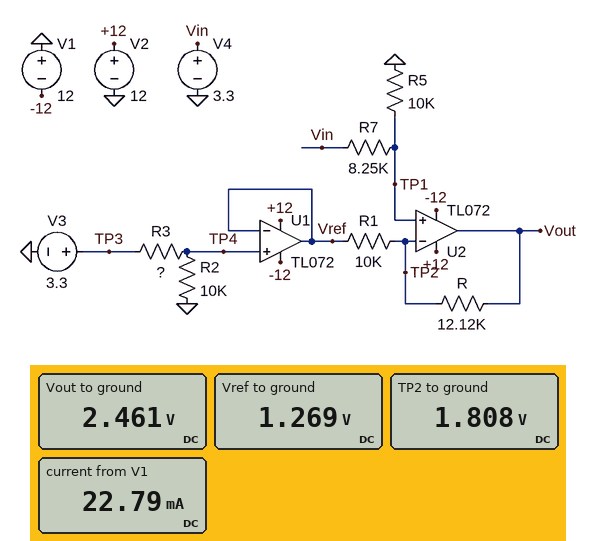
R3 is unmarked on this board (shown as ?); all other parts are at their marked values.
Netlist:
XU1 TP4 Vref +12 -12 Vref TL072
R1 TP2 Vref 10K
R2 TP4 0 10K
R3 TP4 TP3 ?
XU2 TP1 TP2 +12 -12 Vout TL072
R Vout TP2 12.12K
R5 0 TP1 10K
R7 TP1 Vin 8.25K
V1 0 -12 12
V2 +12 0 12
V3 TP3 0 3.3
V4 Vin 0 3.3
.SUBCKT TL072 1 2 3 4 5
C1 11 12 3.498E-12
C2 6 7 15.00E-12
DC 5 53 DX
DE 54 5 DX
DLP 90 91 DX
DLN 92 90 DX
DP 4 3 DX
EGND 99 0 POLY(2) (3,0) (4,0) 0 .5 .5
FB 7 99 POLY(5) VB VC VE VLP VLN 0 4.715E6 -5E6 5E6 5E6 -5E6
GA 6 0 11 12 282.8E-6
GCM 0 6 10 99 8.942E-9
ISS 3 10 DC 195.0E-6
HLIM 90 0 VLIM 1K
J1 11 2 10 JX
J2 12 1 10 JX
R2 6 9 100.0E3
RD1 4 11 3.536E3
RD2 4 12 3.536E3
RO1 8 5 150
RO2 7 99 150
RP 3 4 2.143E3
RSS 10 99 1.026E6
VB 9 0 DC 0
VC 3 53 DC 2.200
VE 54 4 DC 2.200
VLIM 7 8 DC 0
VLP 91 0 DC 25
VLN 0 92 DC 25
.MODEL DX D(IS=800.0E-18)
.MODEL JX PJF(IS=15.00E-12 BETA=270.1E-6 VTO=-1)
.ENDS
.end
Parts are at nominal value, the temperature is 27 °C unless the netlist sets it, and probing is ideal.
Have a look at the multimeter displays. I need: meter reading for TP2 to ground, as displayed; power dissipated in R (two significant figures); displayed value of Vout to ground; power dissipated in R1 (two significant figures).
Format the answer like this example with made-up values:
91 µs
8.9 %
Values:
1.808 V
35 µW
2.461 V
29 µW
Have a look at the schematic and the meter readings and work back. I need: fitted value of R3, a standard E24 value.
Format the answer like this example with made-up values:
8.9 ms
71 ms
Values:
16 kΩ
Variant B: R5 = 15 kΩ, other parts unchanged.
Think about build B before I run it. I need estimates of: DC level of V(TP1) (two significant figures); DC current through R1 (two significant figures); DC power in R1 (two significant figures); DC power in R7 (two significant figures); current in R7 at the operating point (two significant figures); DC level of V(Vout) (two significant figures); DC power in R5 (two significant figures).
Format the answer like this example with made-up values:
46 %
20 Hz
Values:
2.1 V
86 µA
74 µW
170 µW
140 µA
3.2 V
300 µW
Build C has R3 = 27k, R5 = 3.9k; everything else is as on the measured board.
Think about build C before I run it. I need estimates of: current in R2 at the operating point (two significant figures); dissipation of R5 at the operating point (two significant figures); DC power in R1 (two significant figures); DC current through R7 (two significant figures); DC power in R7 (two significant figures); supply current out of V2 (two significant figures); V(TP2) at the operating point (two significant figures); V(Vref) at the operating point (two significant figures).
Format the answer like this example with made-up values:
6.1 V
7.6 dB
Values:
89 µA
290 µW
2.8 µW
270 µA
610 µW
23 mA
1.1 V
890 mV
